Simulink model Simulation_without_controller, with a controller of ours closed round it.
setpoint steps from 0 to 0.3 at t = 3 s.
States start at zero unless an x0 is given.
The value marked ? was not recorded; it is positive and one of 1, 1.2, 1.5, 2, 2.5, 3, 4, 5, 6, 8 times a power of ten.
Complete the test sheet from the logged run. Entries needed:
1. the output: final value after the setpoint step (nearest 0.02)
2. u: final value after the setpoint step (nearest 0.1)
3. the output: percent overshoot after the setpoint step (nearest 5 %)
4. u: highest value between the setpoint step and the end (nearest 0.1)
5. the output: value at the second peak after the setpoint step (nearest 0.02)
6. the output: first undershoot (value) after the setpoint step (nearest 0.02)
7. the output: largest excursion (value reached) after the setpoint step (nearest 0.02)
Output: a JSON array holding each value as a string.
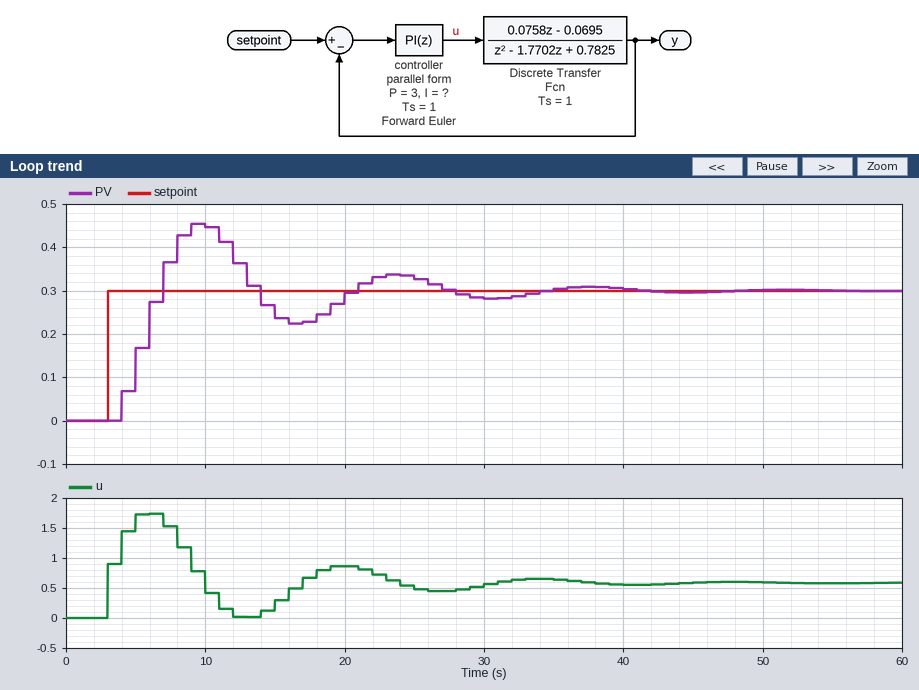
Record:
["0.30", "0.6", "50 %", "1.7", "0.34", "0.22", "0.46"]
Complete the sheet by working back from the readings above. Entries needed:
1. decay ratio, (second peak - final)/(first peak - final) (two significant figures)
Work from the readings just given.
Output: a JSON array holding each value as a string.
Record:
["0.25"]
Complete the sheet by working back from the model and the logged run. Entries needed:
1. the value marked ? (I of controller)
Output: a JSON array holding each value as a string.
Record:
["2.5"]
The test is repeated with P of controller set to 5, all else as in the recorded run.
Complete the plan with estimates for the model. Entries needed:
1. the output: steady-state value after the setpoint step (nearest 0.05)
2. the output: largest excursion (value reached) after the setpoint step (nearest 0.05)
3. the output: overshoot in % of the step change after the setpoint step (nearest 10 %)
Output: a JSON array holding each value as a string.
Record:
["0.30", "0.40", "30 %"]
